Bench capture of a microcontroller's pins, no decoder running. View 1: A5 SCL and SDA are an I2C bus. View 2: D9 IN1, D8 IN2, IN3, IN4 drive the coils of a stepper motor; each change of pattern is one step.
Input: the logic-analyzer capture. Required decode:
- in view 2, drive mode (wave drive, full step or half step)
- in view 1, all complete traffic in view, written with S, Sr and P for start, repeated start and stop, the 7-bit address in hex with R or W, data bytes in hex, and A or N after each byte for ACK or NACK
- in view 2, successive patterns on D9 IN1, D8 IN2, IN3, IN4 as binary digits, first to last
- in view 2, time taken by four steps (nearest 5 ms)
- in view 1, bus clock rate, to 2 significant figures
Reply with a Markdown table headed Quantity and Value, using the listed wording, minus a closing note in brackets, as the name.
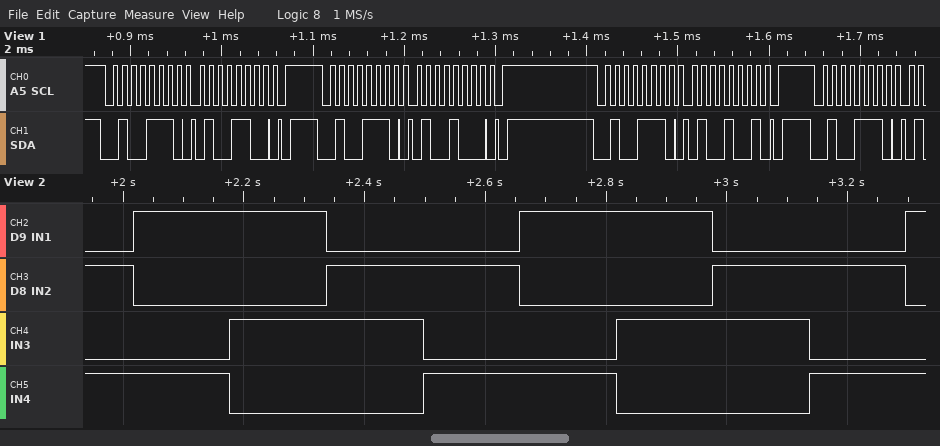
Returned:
| Quantity | Value |
|---|---|
| in view 2, drive mode | full step |
| in view 1, all complete traffic in view, written with S, Sr and P for start, repeated start and stop, the 7-bit address in hex with R or W, data bytes in hex, and A or N after each byte for ACK or NACK | S 27W A 4C A P S 27W A 48 A P S 27W A 49 A P S 27W A |
| in view 2, successive patterns on D9 IN1, D8 IN2, IN3, IN4 as binary digits, first to last | 0101 1001 1010 0110 0101 1001 1010 0110 0101 1001 |
| in view 2, time taken by four steps | 640 ms |
| in view 1, bus clock rate, to 2 significant figures | 100 kHz |
